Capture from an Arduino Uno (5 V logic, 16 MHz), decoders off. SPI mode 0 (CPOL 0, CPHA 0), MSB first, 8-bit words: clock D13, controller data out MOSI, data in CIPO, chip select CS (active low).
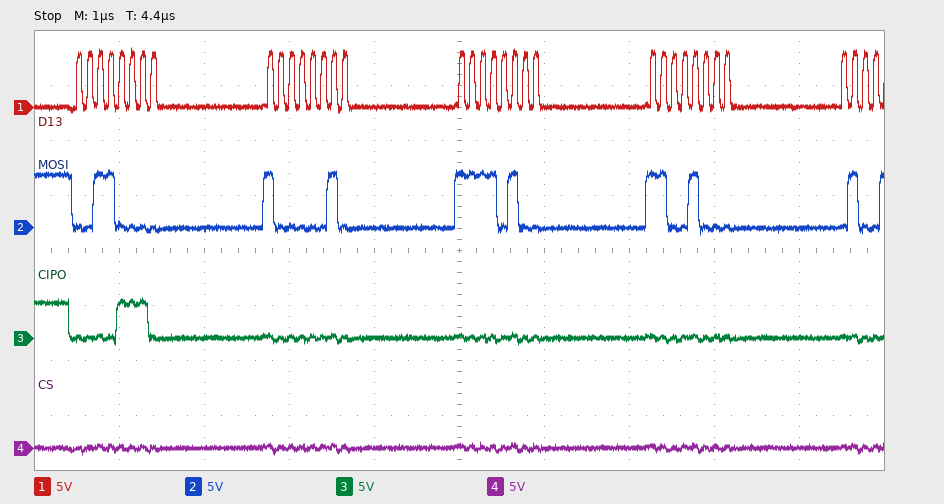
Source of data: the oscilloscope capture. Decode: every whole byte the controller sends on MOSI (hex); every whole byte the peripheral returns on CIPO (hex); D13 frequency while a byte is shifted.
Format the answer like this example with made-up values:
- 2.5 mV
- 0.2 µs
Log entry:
- 0x30 0x82 0xF4 0xC8
- 0x0E 0x00 0x00 0x00
- 8 MHz
